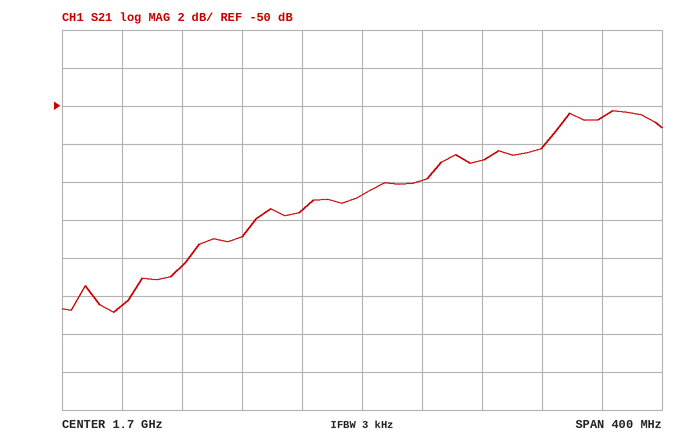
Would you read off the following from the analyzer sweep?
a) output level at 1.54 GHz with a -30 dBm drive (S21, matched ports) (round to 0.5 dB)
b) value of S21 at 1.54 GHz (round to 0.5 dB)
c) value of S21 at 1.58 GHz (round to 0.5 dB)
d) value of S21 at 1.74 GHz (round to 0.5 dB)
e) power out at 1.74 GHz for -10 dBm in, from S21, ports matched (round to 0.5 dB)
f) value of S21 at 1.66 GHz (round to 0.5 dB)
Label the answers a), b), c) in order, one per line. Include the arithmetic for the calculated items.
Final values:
a) -30 dBm + (-60.5 dB) = -90.5 dBm
b) -60.5 dB
c) -58.5 dB
d) -54.0 dB
e) -10 dBm + (-54.0 dB) = -64.0 dBm
f) -55.5 dB
